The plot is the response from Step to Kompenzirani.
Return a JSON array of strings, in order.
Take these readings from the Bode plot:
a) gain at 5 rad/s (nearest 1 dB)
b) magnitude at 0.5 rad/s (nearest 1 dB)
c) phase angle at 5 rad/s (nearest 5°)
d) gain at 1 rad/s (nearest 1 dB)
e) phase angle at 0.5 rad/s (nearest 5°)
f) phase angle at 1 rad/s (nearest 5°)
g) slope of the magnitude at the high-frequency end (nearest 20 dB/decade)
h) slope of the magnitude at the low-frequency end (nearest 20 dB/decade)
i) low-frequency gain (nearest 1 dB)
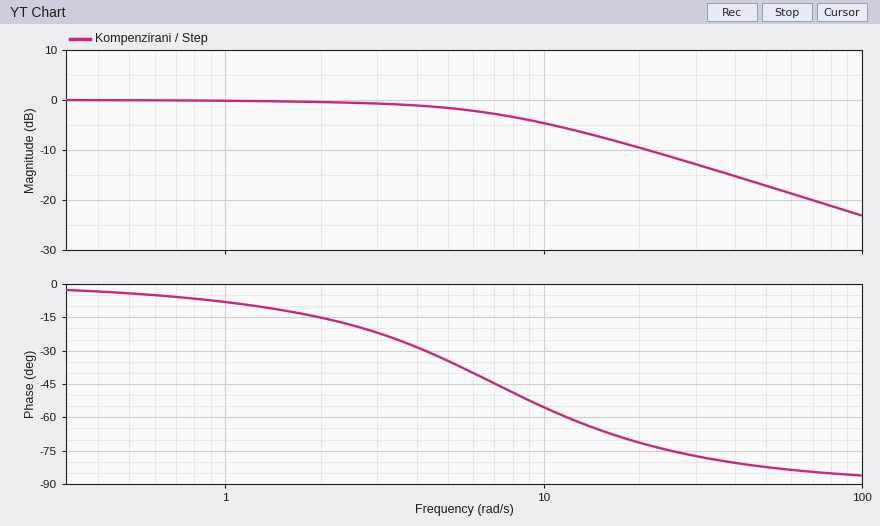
["-2 dB", "0 dB", "-35°", "0 dB", "-5°", "-10°", "-20 dB/decade", "0 dB/decade", "0 dB"]
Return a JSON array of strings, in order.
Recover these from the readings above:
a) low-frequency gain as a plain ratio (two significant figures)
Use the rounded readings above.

["1.0"]
